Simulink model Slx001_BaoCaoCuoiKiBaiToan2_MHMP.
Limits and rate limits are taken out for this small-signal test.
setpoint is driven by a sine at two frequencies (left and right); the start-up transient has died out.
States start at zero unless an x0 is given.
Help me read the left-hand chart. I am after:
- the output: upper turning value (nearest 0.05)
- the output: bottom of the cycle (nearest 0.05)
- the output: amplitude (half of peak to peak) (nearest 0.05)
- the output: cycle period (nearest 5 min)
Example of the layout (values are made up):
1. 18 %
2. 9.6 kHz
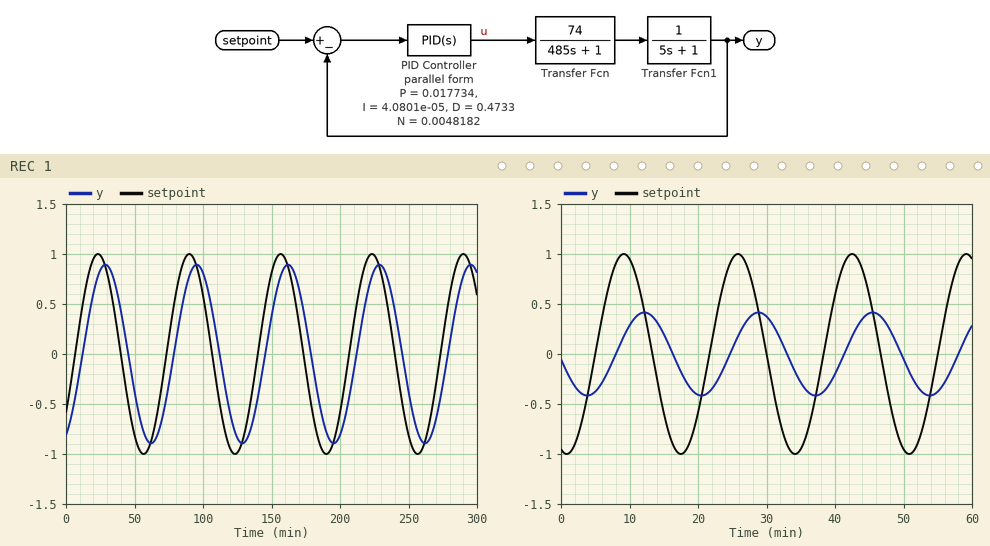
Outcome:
1. 0.90
2. -0.90
3. 0.90
4. 65 min
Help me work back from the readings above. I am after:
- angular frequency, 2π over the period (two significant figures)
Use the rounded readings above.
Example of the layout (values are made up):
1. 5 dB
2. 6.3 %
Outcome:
1. 0.097 rad/min
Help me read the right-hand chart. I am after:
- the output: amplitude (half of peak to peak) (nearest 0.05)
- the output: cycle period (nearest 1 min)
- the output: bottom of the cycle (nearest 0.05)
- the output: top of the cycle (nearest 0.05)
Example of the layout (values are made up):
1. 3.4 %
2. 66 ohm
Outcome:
1. 0.40
2. 17 min
3. -0.40
4. 0.40
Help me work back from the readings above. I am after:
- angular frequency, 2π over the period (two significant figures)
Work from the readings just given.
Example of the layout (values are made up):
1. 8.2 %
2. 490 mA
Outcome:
1. 0.37 rad/min
